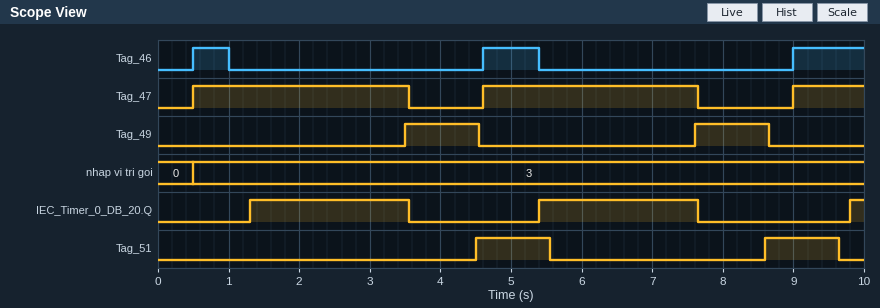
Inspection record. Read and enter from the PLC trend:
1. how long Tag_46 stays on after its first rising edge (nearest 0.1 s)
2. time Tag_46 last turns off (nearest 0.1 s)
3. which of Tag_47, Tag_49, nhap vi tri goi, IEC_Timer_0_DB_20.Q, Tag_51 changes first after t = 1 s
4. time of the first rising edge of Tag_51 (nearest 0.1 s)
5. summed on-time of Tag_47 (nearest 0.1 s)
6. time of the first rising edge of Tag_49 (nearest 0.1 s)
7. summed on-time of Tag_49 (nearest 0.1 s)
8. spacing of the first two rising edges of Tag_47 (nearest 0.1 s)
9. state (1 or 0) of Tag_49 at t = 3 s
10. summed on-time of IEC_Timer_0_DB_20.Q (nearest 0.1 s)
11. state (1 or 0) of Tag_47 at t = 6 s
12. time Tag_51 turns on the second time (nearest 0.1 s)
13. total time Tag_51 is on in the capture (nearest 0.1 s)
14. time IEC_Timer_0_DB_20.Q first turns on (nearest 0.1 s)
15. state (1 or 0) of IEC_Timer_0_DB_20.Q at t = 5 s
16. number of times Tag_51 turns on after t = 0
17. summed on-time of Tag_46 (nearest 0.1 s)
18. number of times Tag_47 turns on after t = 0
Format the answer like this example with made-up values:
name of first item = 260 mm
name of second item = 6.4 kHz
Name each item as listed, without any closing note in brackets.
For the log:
how long Tag_46 stays on after its first rising edge = 0.5 s
time Tag_46 last turns off = 5.4 s
which of Tag_47, Tag_49, nhap vi tri goi, IEC_Timer_0_DB_20.Q, Tag_51 changes first after t = 1 s = IEC_Timer_0_DB_20.Q
time of the first rising edge of Tag_51 = 4.5 s
summed on-time of Tag_47 = 7.1 s
time of the first rising edge of Tag_49 = 3.5 s
summed on-time of Tag_49 = 2.1 s
spacing of the first two rising edges of Tag_47 = 4.1 s
state (1 or 0) of Tag_49 at t = 3 s = 0
summed on-time of IEC_Timer_0_DB_20.Q = 4.7 s
state (1 or 0) of Tag_47 at t = 6 s = 1
time Tag_51 turns on the second time = 8.6 s
total time Tag_51 is on in the capture = 2.1 s
time IEC_Timer_0_DB_20.Q first turns on = 1.3 s
state (1 or 0) of IEC_Timer_0_DB_20.Q at t = 5 s = 0
number of times Tag_51 turns on after t = 0 = 2
summed on-time of Tag_46 = 2.3 s
number of times Tag_47 turns on after t = 0 = 3
